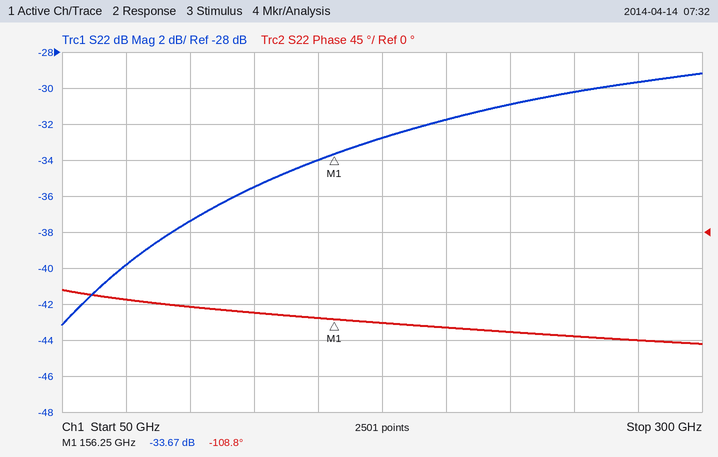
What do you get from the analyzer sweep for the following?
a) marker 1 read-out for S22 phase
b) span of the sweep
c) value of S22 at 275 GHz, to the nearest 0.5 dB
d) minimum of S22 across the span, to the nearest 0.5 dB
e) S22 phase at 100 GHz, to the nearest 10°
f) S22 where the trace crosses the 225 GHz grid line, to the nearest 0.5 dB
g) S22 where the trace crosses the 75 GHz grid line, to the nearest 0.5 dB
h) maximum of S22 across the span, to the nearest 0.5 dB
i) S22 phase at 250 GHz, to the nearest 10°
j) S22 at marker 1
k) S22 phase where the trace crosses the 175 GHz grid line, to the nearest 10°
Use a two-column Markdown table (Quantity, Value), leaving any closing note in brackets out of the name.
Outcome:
| Quantity | Value |
|---|---|
| marker 1 read-out for S22 phase | -108.8° |
| span of the sweep | 250 GHz |
| value of S22 at 275 GHz, to the nearest 0.5 dB | -29.5 dB |
| minimum of S22 across the span, to the nearest 0.5 dB | -43.0 dB |
| S22 phase at 100 GHz, to the nearest 10° | -90° |
| S22 where the trace crosses the 225 GHz grid line, to the nearest 0.5 dB | -31.0 dB |
| S22 where the trace crosses the 75 GHz grid line, to the nearest 0.5 dB | -40.0 dB |
| maximum of S22 across the span, to the nearest 0.5 dB | -29.0 dB |
| S22 phase at 250 GHz, to the nearest 10° | -130° |
| S22 at marker 1 | -33.67 dB |
| S22 phase where the trace crosses the 175 GHz grid line, to the nearest 10° | -110° |
